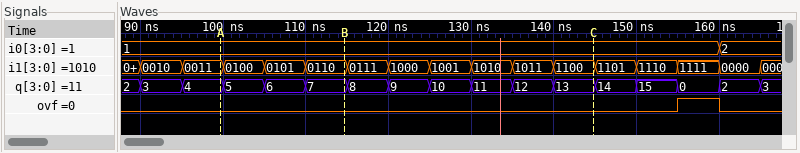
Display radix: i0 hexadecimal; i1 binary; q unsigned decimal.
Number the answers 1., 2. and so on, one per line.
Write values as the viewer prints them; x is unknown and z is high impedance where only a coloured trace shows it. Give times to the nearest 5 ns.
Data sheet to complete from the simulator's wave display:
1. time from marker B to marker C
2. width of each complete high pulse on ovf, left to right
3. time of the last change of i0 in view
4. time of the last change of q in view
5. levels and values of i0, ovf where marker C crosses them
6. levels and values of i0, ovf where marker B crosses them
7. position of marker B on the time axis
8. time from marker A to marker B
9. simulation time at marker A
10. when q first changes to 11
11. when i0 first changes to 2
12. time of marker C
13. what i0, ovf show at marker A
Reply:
1. 30 ns
2. 5 ns
3. 160 ns
4. 165 ns
5. i0=1, ovf=0
6. i0=1, ovf=0
7. 115 ns
8. 15 ns
9. 100 ns
10. 130 ns
11. 160 ns
12. 145 ns
13. i0=1, ovf=0
